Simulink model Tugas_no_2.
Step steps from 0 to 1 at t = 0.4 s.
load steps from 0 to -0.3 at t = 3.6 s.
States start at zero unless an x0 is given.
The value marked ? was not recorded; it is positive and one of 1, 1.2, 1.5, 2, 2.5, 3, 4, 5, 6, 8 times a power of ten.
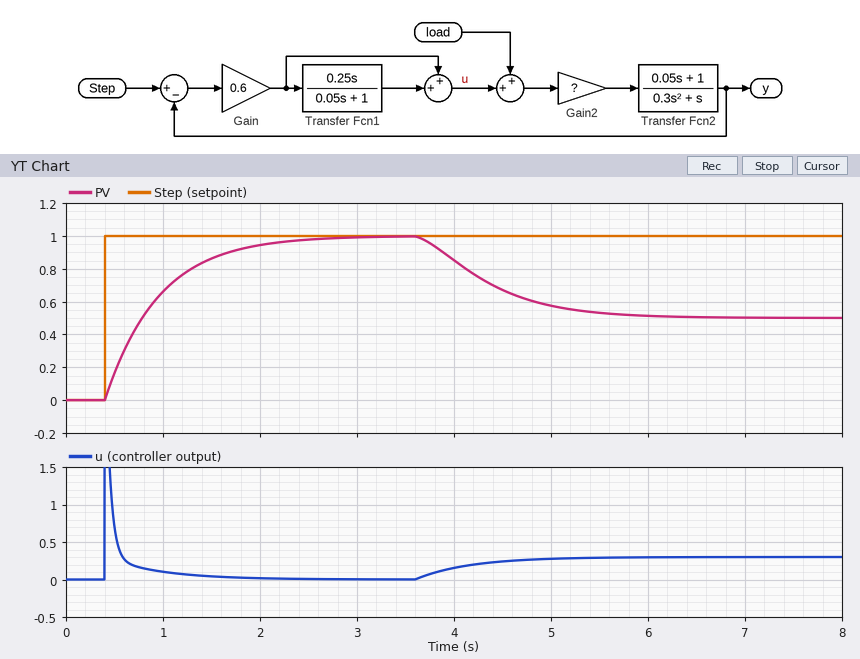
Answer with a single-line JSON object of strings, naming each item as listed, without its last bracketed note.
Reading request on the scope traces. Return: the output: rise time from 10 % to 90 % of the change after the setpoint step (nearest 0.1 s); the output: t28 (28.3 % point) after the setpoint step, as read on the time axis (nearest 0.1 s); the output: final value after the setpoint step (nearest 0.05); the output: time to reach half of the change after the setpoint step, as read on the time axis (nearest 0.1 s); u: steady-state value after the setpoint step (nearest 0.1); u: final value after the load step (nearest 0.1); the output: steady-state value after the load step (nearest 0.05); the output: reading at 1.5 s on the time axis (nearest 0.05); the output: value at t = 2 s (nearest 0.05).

{"the output: rise time from 10 % to 90 % of the change after the setpoint step": "1.2 s", "the output: t28 (28.3 % point) after the setpoint step, as read on the time axis": "0.6 s", "the output: final value after the setpoint step": "1.00", "the output: time to reach half of the change after the setpoint step, as read on the time axis": "0.8 s", "u: steady-state value after the setpoint step": "0.0", "u: final value after the load step": "0.3", "the output: steady-state value after the load step": "0.50", "the output: reading at 1.5 s on the time axis": "0.85", "the output: value at t = 2 s": "0.95"}
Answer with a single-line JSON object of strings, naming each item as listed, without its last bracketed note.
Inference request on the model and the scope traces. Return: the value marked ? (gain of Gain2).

{"the value marked ?": "3"}
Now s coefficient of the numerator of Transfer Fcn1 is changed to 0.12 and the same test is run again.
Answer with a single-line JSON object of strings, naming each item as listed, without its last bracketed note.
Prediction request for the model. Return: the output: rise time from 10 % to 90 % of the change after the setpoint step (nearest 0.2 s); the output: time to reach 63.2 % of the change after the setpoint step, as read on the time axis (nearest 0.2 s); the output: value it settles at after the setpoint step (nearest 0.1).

{"the output: rise time from 10 % to 90 % of the change after the setpoint step": "1.0 s", "the output: time to reach 63.2 % of the change after the setpoint step, as read on the time axis": "1.0 s", "the output: value it settles at after the setpoint step": "1.0"}
